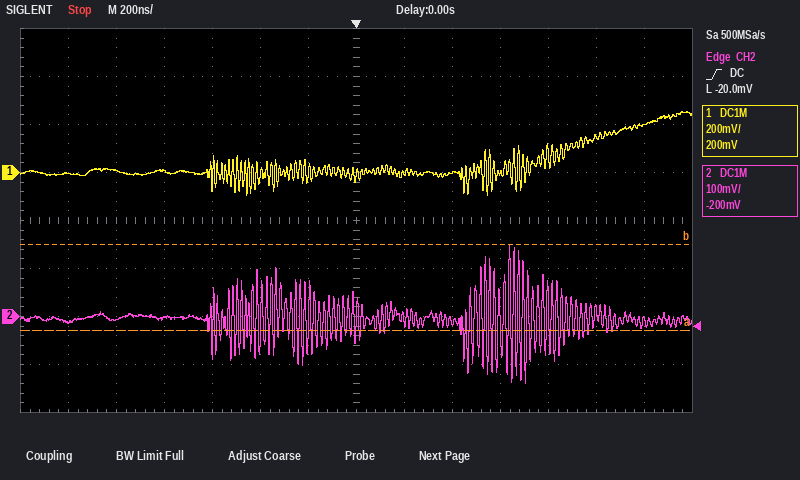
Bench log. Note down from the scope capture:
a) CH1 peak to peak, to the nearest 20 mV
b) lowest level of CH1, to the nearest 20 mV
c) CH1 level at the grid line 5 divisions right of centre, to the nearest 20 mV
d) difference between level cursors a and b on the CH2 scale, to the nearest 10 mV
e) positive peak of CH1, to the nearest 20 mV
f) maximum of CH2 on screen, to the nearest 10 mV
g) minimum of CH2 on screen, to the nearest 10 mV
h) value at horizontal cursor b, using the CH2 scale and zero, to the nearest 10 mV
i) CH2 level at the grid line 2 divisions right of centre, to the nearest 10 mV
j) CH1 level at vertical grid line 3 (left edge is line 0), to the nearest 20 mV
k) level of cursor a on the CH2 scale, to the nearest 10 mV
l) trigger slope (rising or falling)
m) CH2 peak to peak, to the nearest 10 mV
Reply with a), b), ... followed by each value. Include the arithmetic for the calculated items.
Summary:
a) 260 mV − (-100 mV) = 360 mV
b) -100 mV
c) 140 mV
d) 180 mV
e) 260 mV
f) 150 mV
g) -140 mV
h) 150 mV
i) -10 mV
j) 0 mV
k) -30 mV
l) rising
m) 150 mV − (-140 mV) = 290 mV
